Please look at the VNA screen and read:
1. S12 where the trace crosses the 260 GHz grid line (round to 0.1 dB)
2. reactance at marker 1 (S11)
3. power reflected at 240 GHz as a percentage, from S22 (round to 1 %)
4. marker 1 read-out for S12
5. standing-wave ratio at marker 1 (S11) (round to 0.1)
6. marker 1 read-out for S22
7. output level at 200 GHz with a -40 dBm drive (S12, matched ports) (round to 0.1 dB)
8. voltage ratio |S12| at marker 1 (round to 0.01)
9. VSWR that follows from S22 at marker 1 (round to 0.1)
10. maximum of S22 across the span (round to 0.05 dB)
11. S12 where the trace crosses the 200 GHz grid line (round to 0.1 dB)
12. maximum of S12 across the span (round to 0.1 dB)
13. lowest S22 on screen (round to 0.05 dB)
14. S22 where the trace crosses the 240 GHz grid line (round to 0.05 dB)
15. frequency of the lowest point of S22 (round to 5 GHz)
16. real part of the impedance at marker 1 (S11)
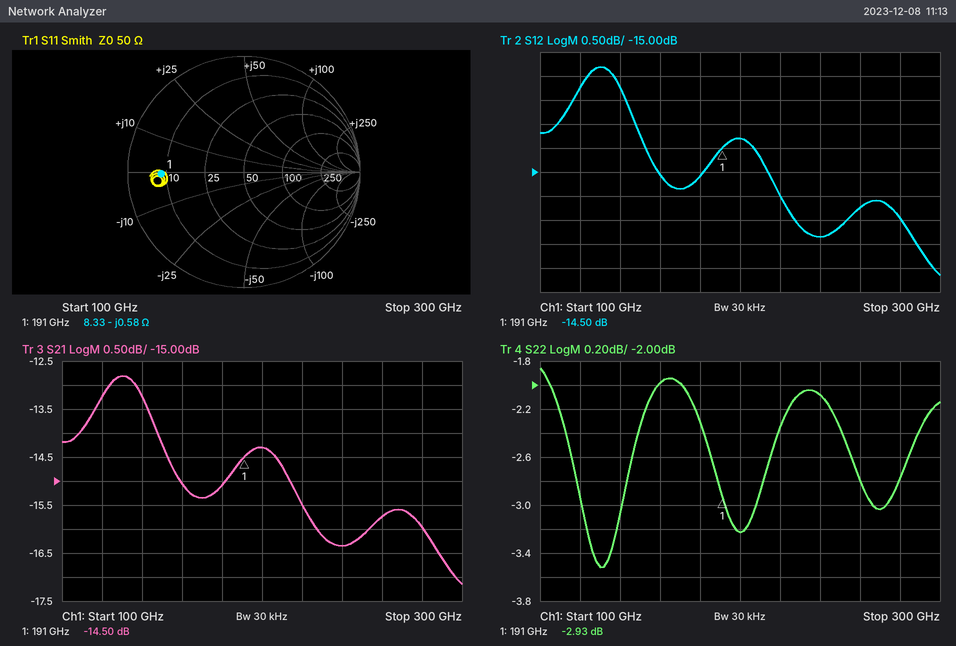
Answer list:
-15.7 dB
-0.58 Ω
62 %
-14.50 dB
6.0
-2.93 dB
-54.3 dBm
0.19
6.0
-1.85 dB
-14.3 dB
-12.8 dB
-3.50 dB
-2.10 dB
130 GHz
8.33 Ω
